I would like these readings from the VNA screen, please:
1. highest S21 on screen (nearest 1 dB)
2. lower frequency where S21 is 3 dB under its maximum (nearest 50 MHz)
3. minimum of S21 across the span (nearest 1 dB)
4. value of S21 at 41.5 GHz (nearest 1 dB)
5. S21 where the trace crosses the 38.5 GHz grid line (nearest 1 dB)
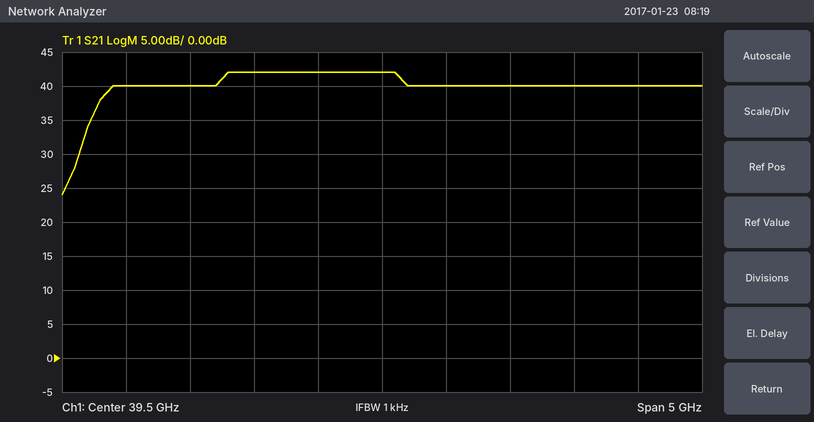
42 dB
37.35 GHz
24 dB
40 dB
42 dB
